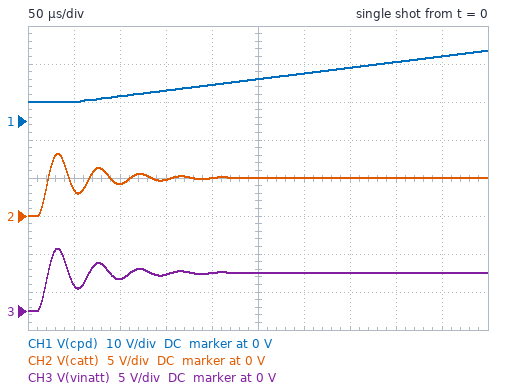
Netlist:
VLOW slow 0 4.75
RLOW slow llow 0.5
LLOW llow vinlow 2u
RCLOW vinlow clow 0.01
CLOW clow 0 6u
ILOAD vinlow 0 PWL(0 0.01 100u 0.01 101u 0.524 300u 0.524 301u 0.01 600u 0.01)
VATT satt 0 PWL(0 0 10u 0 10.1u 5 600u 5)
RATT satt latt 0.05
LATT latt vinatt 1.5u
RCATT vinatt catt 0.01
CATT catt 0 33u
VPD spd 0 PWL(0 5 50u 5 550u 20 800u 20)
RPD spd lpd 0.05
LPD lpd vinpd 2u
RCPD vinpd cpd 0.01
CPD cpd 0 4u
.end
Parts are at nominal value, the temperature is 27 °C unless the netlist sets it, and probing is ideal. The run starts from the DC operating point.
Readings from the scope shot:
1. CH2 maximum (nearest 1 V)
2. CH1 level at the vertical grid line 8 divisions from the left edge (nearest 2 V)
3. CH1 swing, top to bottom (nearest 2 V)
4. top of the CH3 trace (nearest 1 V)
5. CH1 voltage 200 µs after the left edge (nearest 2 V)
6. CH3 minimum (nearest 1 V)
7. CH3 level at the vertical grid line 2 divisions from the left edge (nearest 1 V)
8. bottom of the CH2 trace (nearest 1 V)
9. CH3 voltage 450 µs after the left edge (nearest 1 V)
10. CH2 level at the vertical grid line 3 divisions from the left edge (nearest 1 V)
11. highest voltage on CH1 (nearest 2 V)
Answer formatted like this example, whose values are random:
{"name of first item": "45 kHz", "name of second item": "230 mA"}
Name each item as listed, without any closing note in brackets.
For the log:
{"CH2 maximum": "8 V", "CH1 level at the vertical grid line 8 divisions from the left edge": "16 V", "CH1 swing, top to bottom": "14 V", "top of the CH3 trace": "8 V", "CH1 voltage 200 µs after the left edge": "10 V", "CH3 minimum": "0 V", "CH3 level at the vertical grid line 2 divisions from the left edge": "4 V", "bottom of the CH2 trace": "0 V", "CH3 voltage 450 µs after the left edge": "5 V", "CH2 level at the vertical grid line 3 divisions from the left edge": "5 V", "highest voltage on CH1": "18 V"}
